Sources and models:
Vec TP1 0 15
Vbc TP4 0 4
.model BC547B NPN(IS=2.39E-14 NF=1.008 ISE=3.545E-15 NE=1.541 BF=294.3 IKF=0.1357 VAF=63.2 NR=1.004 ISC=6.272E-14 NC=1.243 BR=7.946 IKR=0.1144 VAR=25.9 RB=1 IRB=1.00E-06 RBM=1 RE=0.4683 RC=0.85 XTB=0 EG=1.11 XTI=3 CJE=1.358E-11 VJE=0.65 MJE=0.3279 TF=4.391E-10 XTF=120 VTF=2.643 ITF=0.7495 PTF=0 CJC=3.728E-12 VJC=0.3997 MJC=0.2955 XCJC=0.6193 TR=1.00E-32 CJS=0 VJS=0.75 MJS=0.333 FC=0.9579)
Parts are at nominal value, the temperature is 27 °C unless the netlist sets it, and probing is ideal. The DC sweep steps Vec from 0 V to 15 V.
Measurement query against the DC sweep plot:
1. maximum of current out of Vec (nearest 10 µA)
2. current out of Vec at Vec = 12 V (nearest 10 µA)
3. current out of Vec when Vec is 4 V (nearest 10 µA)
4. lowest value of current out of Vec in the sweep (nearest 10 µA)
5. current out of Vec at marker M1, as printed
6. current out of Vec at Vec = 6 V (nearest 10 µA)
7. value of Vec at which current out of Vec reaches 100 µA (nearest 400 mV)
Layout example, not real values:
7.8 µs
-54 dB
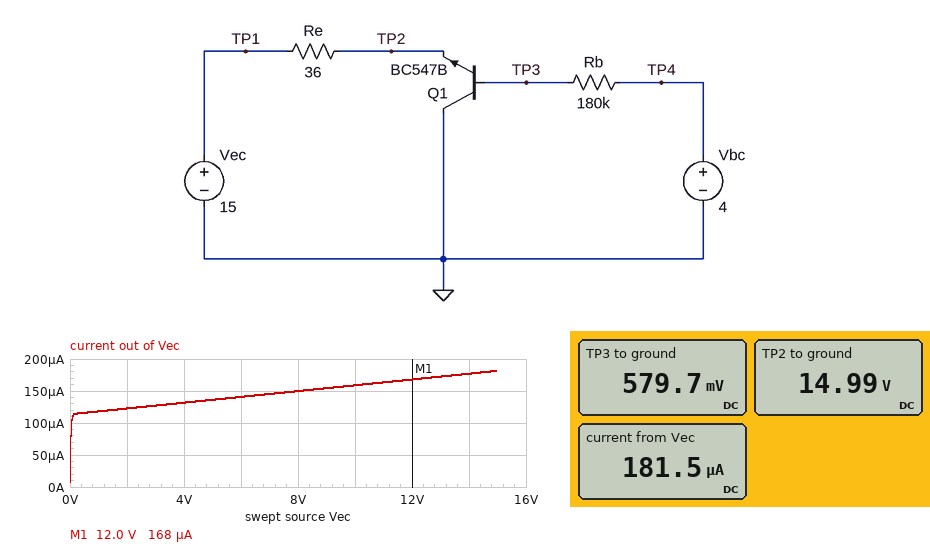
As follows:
180 µA
170 µA
130 µA
10 µA
168 µA
140 µA
0 V
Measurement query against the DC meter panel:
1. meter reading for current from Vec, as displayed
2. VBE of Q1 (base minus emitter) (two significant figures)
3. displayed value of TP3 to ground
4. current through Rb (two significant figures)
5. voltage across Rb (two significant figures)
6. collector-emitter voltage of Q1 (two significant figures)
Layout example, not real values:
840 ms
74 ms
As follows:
181.5 µA
-14 V
579.7 mV
19 µA
3.4 V
-15 V
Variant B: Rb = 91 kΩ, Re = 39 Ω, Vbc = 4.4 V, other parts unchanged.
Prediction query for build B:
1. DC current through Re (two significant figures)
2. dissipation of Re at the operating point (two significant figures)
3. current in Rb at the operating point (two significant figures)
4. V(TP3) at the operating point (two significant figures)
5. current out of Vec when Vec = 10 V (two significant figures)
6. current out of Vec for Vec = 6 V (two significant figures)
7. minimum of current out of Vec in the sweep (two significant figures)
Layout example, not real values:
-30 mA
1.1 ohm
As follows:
410 µA
6.6 µW
42 µA
600 mV
360 µA
320 µA
15 µA
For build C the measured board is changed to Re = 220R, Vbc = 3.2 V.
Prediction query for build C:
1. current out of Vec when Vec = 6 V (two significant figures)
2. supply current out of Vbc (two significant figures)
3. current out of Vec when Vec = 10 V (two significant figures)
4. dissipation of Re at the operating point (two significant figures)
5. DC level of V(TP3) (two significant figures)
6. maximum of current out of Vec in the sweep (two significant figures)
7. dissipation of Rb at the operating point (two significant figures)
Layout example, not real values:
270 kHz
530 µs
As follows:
110 µA
15 µA
120 µA
4.2 µW
570 mV
140 µA
38 µW
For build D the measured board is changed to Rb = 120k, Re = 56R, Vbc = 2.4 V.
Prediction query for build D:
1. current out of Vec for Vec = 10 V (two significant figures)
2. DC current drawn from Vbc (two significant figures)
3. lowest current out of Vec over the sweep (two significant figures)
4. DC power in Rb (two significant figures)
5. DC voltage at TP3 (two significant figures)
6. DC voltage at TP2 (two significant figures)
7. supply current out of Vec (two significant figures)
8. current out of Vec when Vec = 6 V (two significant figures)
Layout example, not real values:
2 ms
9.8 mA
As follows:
130 µA
15 µA
6.0 µA
28 µW
570 mV
15 V
140 µA
110 µA
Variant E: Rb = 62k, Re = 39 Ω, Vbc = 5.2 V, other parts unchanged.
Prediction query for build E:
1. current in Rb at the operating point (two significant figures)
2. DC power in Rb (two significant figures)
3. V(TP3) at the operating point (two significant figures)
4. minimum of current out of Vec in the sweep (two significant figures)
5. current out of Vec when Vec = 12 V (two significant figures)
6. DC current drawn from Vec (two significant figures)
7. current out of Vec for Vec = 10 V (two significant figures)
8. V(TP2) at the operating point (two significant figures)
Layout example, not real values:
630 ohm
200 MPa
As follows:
74 µA
340 µW
620 mV
23 µA
690 µA
740 µA
650 µA
15 V
